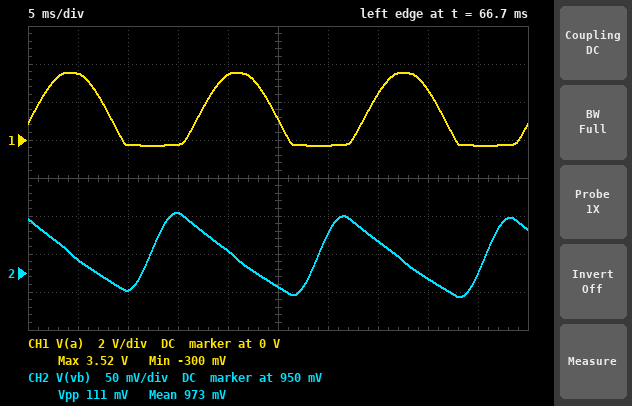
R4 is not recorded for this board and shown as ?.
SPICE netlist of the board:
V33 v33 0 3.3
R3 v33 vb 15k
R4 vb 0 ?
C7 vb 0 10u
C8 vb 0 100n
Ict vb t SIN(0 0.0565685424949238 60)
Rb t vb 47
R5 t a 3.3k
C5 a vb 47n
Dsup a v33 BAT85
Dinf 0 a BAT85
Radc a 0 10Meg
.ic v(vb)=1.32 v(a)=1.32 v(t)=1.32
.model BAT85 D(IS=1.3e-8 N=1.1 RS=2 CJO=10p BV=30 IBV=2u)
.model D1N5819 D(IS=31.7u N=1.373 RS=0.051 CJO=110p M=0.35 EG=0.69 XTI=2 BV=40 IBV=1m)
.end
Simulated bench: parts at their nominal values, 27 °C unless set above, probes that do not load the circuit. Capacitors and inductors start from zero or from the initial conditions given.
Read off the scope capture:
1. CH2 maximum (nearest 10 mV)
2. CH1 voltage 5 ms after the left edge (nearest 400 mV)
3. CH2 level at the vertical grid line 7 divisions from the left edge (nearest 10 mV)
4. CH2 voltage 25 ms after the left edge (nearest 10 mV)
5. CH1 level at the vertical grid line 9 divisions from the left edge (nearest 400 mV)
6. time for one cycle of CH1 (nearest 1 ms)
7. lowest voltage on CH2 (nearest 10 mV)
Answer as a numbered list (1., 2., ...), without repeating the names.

1. 1.03 V
2. 3.6 V
3. 990 mV
4. 930 mV
5. -400 mV
6. 17 ms
7. 920 mV
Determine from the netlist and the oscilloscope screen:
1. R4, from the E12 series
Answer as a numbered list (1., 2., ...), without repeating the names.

1. 3.9 kΩ
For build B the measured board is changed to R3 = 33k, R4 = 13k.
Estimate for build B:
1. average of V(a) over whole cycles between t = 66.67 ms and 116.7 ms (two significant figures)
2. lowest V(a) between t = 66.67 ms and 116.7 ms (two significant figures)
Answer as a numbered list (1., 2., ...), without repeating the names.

1. 1.5 V
2. -290 mV
